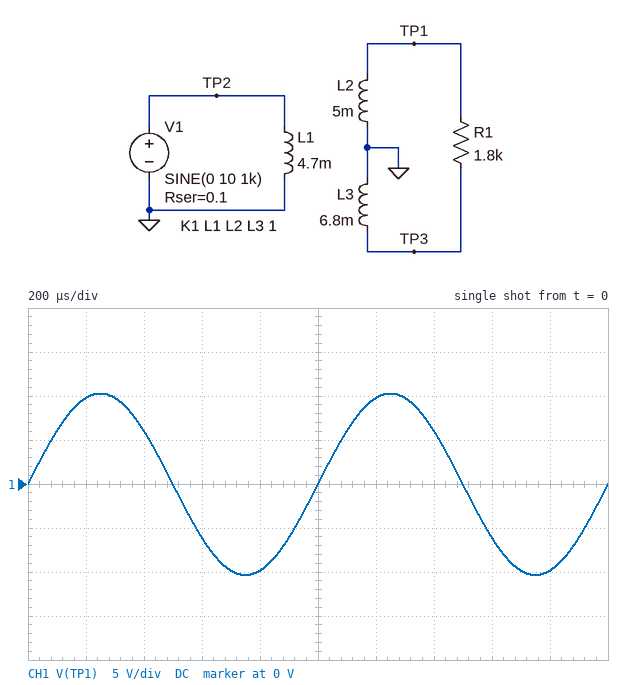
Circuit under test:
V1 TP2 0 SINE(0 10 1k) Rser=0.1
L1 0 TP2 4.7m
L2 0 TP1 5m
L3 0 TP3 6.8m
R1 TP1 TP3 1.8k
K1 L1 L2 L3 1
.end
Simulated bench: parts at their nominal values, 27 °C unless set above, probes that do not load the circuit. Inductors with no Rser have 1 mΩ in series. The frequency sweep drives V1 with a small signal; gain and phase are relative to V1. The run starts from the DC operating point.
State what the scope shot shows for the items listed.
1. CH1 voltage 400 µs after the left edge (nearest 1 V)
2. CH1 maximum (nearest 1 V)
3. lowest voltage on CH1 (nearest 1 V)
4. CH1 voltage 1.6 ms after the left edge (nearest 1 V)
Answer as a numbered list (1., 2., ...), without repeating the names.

1. 6 V
2. 10 V
3. -10 V
4. -6 V
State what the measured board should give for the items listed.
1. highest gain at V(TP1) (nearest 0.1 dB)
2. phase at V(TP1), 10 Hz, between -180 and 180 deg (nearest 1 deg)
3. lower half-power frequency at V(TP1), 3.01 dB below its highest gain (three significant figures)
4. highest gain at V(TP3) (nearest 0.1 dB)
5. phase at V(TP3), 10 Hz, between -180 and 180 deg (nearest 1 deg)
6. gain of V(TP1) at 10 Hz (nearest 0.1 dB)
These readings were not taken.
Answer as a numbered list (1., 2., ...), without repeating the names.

1. 0.3 dB
2. 19 deg
3. 3.42 Hz
4. 1.6 dB
5. 19 deg
6. -0.2 dB
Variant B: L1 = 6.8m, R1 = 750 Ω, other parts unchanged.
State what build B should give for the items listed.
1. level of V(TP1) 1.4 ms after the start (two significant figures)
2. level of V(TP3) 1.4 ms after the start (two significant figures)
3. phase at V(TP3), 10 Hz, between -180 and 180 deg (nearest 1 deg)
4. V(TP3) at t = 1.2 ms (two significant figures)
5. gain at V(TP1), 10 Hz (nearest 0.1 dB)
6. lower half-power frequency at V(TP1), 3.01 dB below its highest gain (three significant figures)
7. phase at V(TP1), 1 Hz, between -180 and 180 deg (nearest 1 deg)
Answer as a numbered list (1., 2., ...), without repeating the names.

1. 5.0 V
2. 5.8 V
3. 13 deg
4. 9.5 V
5. -1.6 dB
6. 2.36 Hz
7. 67 deg
